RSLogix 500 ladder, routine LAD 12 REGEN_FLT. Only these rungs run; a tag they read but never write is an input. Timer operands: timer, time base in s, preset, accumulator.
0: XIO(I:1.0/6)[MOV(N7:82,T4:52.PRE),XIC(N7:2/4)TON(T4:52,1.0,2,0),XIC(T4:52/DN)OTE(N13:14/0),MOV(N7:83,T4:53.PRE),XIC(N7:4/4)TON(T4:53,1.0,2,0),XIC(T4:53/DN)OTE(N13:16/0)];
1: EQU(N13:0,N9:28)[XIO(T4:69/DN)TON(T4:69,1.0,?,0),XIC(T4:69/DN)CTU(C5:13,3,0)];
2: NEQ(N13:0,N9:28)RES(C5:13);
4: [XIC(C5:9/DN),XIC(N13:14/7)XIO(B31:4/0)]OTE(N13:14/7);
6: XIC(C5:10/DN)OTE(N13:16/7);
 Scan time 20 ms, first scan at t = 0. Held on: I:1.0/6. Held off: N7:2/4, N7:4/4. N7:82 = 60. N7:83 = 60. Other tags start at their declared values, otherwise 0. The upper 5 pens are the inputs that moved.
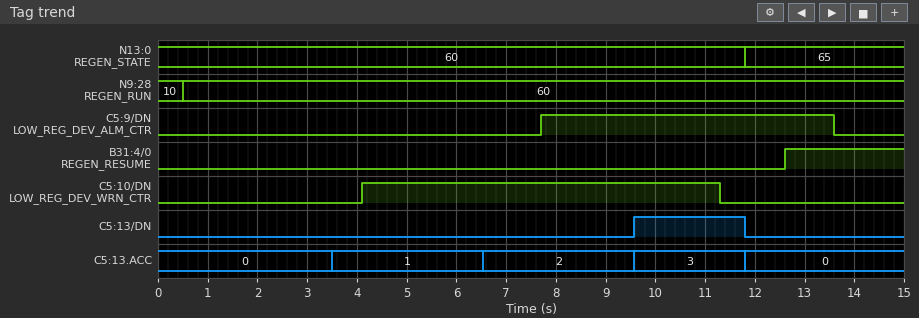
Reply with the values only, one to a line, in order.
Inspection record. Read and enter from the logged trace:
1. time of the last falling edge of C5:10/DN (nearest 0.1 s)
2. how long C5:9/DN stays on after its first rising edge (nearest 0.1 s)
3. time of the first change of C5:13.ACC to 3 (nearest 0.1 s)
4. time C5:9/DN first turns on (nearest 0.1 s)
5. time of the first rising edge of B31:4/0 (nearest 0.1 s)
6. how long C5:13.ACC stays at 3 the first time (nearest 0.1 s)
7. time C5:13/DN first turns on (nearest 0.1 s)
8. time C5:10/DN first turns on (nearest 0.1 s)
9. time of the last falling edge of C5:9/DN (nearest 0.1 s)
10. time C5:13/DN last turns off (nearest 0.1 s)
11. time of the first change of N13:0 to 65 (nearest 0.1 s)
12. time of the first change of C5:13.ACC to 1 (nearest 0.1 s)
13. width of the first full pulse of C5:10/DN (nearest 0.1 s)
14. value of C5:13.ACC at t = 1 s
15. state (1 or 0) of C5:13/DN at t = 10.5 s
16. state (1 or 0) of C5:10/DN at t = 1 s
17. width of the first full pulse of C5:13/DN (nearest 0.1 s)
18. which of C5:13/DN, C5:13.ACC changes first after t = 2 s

11.3 s
5.9 s
9.6 s
7.7 s
12.6 s
2.2 s
9.6 s
4.1 s
13.6 s
11.8 s
11.8 s
3.5 s
7.2 s
0
1
0
2.2 s
C5:13.ACC
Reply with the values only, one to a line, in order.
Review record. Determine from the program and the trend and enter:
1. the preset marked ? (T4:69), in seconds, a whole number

3 s
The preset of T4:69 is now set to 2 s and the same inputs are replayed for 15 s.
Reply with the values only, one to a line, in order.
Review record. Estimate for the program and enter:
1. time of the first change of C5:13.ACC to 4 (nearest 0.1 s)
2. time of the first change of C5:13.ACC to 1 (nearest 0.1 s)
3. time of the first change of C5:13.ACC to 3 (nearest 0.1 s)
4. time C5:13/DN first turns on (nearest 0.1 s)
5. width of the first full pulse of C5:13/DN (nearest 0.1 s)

8.6 s
2.5 s
6.6 s
6.6 s
5.2 s
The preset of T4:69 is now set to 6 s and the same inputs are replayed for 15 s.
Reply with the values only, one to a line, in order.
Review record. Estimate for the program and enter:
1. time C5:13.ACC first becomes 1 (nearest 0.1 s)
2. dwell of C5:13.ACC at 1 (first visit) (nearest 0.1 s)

6.5 s
5.3 s
